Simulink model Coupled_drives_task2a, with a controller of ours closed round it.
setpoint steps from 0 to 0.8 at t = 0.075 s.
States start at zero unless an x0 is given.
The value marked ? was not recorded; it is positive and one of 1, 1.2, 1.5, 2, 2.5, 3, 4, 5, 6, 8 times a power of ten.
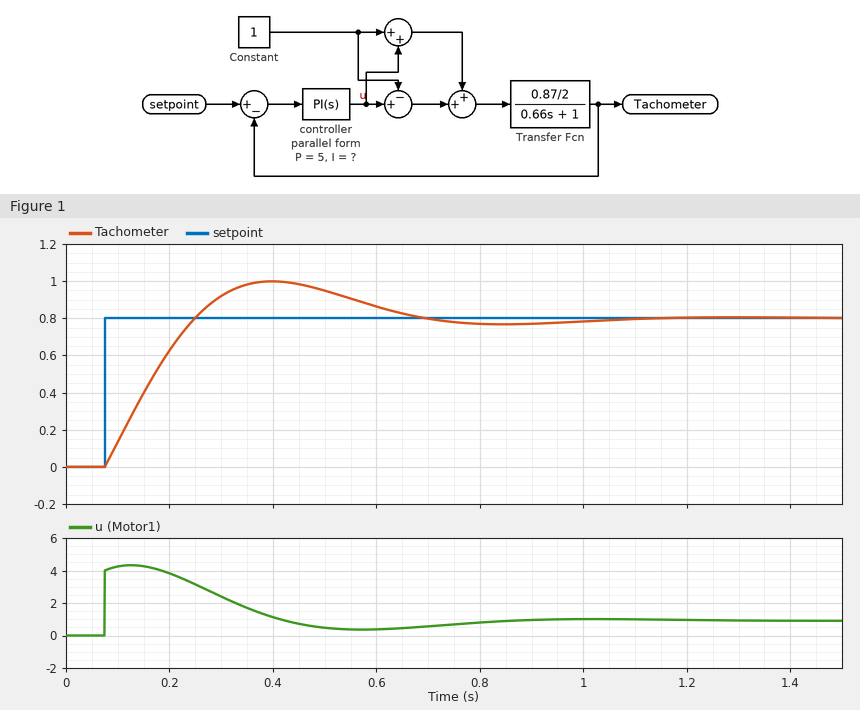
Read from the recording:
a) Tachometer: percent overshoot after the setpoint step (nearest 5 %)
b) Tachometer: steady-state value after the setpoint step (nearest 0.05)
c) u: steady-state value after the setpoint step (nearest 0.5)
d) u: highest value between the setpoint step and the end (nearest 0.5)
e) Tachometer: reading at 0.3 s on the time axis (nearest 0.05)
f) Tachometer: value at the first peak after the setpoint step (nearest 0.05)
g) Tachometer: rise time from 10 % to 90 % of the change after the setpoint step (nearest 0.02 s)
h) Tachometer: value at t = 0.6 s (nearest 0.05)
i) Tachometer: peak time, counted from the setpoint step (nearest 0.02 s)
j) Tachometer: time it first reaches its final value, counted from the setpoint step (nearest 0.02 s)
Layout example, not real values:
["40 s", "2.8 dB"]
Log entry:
["25 %", "0.80", "1.0", "4.5", "0.90", "1.00", "0.14 s", "0.85", "0.32 s", "0.18 s"]
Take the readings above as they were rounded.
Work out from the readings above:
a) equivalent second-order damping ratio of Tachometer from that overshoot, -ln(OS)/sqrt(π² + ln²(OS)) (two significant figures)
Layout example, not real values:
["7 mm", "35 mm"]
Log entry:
["0.40"]
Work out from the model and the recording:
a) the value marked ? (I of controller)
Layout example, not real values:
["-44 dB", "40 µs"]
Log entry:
["50"]
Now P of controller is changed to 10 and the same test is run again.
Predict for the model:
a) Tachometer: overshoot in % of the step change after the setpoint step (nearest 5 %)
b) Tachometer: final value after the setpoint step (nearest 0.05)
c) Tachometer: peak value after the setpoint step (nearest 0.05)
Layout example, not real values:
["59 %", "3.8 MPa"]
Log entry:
["10 %", "0.80", "0.90"]
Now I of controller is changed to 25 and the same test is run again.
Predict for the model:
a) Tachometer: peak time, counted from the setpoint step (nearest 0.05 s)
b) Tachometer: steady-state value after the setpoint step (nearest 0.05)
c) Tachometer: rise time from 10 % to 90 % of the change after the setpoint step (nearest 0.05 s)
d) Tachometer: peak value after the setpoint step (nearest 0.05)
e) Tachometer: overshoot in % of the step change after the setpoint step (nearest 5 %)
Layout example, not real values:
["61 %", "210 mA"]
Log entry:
["0.45 s", "0.80", "0.20 s", "0.90", "15 %"]
